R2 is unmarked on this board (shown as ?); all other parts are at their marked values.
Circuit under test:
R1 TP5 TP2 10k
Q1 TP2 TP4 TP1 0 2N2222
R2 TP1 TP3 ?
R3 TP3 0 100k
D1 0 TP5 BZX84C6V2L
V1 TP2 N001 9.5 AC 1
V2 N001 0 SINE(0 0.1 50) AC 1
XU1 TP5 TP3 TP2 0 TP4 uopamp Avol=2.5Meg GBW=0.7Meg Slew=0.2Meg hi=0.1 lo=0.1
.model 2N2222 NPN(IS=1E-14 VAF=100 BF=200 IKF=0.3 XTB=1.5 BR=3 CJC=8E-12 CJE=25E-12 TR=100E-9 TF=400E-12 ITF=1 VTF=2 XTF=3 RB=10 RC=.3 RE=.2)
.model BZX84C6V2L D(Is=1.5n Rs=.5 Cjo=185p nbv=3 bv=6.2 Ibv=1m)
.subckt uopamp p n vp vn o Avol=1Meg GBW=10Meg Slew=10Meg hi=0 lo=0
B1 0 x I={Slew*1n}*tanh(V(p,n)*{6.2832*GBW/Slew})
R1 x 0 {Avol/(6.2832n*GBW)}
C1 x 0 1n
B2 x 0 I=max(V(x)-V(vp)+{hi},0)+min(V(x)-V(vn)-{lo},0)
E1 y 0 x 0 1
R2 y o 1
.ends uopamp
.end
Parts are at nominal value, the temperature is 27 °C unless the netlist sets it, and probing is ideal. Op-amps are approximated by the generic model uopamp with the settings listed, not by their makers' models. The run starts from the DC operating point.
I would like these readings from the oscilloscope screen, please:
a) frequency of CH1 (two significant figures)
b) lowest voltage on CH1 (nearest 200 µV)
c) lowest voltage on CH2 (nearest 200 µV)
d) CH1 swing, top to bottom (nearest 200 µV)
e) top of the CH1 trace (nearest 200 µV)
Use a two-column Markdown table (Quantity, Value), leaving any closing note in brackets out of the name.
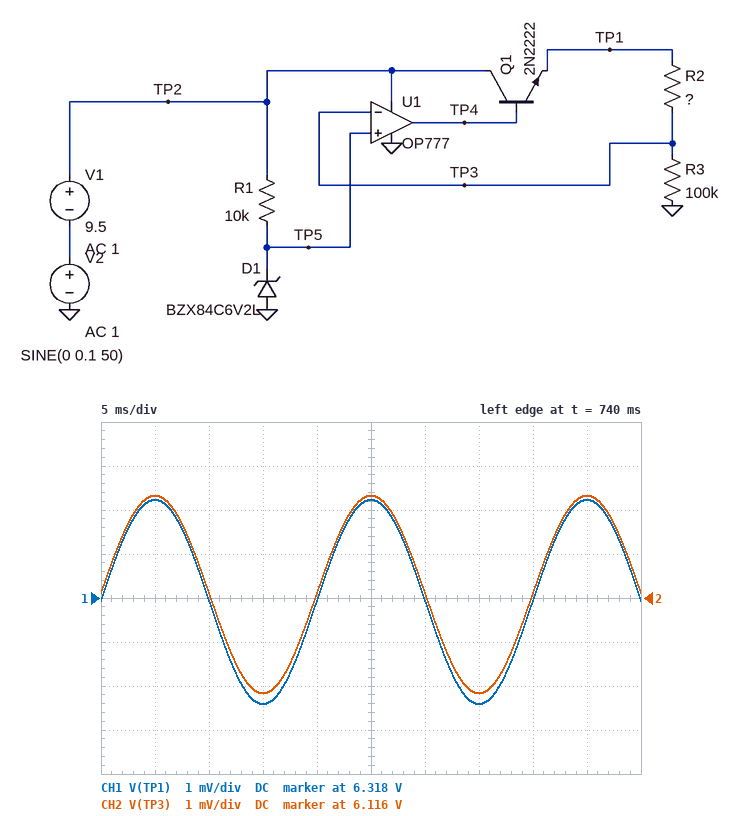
| Quantity | Value |
|---|---|
| frequency of CH1 | 50 Hz |
| lowest voltage on CH1 | 6.3156 V |
| lowest voltage on CH2 | 6.1138 V |
| CH1 swing, top to bottom | 4.6 mV |
| top of the CH1 trace | 6.3202 V |
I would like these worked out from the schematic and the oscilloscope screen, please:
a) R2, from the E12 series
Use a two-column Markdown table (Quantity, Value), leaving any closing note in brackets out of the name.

| Quantity | Value |
|---|---|
| R2, from the E12 series | 3.3 kΩ |
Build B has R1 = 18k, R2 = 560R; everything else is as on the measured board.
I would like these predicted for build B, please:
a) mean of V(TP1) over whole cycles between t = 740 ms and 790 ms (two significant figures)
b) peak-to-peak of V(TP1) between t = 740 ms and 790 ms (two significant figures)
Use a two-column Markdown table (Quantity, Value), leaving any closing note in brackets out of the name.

| Quantity | Value |
|---|---|
| mean of V(TP1) over whole cycles between t = 740 ms and 790 ms | 6.1 V |
| peak-to-peak of V(TP1) between t = 740 ms and 790 ms | 4.5 mV |
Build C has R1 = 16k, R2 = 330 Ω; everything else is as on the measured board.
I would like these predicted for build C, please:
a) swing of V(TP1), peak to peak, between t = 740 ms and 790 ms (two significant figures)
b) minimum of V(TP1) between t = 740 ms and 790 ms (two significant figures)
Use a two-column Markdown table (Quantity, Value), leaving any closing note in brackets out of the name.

| Quantity | Value |
|---|---|
| swing of V(TP1), peak to peak, between t = 740 ms and 790 ms | 4.5 mV |
| minimum of V(TP1) between t = 740 ms and 790 ms | 6.1 V |
